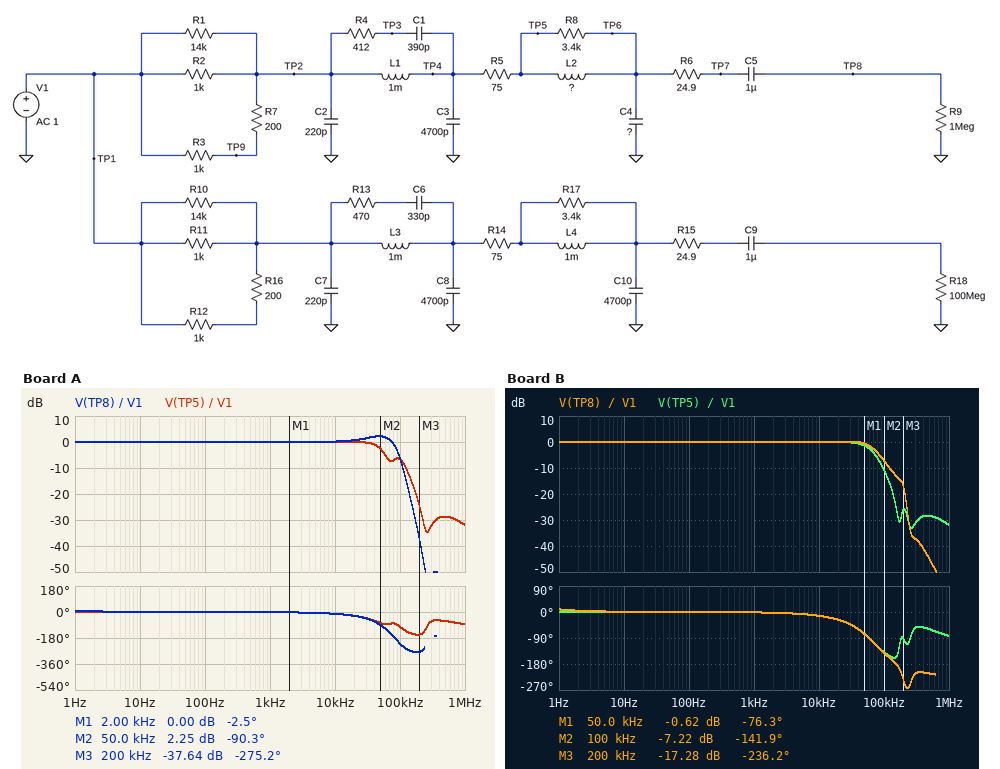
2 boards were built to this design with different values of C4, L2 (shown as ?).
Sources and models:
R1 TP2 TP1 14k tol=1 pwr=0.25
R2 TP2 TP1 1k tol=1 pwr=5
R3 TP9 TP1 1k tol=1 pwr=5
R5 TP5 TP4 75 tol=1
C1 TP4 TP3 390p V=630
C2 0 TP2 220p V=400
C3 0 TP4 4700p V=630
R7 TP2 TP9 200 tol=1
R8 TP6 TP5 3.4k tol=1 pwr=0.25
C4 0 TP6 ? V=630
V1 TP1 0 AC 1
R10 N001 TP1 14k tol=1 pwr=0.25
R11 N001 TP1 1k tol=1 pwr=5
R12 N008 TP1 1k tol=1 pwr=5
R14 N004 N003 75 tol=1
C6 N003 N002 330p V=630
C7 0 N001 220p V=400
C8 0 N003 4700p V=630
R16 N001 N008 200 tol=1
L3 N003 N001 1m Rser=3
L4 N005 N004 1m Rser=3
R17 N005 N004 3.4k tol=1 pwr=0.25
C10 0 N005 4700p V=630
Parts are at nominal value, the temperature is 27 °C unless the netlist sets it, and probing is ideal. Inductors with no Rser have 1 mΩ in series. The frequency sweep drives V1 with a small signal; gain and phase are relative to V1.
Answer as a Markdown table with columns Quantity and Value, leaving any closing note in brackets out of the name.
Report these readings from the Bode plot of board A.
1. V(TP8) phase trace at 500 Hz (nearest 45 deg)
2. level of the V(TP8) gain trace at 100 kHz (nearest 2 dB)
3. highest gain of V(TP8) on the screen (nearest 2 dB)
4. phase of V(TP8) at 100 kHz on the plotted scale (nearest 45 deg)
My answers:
| Quantity | Value |
|---|---|
| V(TP8) phase trace at 500 Hz | 0 deg |
| level of the V(TP8) gain trace at 100 kHz | -6 dB |
| highest gain of V(TP8) on the screen | 2 dB |
| phase of V(TP8) at 100 kHz on the plotted scale | -225 deg |
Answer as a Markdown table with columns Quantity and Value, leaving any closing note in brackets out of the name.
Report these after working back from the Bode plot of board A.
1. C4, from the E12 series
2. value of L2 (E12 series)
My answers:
| Quantity | Value |
|---|---|
| C4, from the E12 series | 1.5 nF |
| value of L2 | 3.3 mH |
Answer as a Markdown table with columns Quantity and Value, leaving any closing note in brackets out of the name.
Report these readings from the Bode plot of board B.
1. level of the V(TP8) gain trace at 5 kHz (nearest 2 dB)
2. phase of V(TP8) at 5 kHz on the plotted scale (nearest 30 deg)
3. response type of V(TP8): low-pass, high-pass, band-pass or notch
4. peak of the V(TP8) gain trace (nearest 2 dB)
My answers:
| Quantity | Value |
|---|---|
| level of the V(TP8) gain trace at 5 kHz | 0 dB |
| phase of V(TP8) at 5 kHz on the plotted scale | 0 deg |
| response type of V(TP8): low-pass, high-pass, band-pass or notch | low-pass |
| peak of the V(TP8) gain trace | 0 dB |
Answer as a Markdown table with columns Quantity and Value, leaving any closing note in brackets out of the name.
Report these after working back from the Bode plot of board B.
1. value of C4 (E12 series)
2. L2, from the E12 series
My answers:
| Quantity | Value |
|---|---|
| value of C4 | 1.8 nF |
| L2, from the E12 series | 470 µH |
